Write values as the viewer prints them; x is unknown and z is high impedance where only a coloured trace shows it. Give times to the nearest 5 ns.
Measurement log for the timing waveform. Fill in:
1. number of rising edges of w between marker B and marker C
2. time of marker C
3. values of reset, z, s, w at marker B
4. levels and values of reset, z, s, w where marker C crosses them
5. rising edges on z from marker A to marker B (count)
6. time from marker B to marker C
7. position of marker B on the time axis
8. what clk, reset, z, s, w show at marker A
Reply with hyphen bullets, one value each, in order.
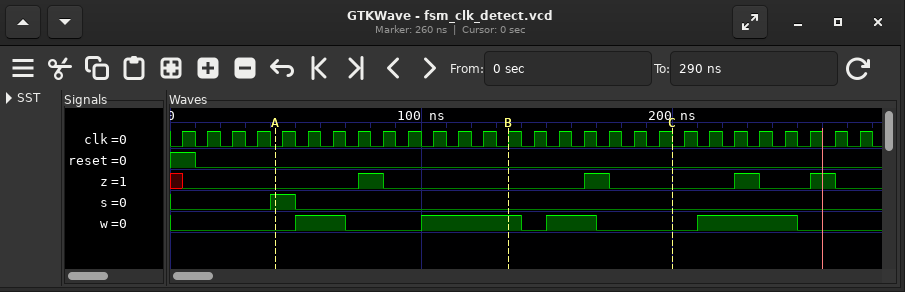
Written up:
- 1
- 200 ns
- reset=0, z=0, s=0, w=1
- reset=0, z=0, s=0, w=0
- 1
- 65 ns
- 135 ns
- clk=0, reset=0, z=0, s=1, w=0
